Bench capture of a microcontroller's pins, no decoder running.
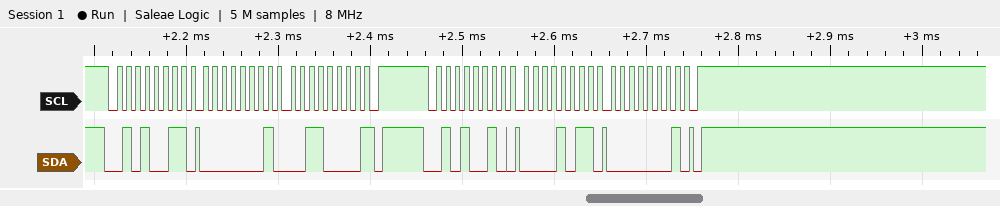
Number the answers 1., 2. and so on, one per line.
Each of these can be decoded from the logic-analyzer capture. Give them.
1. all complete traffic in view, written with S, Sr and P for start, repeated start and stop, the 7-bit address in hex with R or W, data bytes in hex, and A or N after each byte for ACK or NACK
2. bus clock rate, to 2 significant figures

1. S 29R A 01 A 30 N P S 29W A 0B A 01 A P
2. 100 kHz
